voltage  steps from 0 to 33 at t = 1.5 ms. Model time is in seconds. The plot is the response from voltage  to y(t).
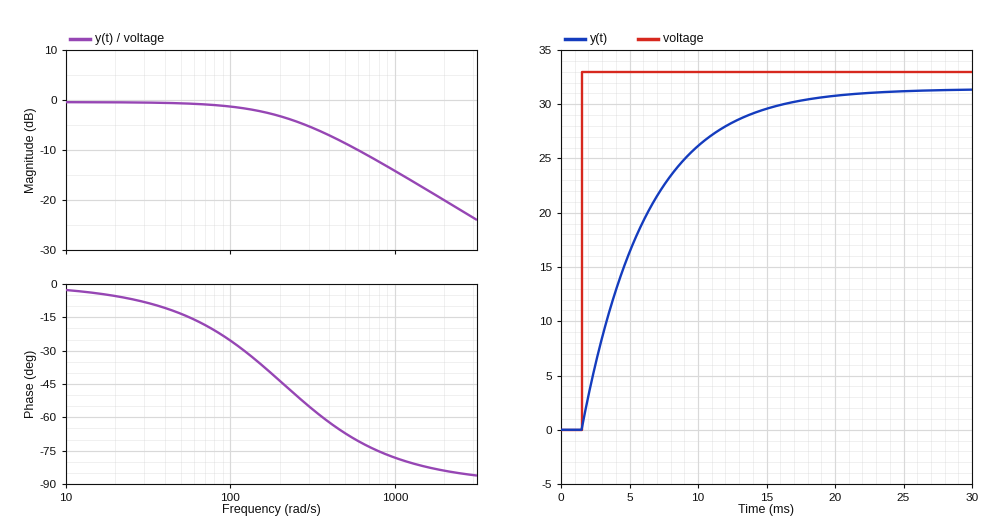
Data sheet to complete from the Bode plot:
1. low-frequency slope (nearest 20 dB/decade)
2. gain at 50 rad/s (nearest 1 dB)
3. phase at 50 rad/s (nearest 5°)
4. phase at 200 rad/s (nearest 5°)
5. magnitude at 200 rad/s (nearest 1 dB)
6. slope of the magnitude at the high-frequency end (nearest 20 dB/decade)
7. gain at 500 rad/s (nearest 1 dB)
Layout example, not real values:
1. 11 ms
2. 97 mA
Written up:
1. 0 dB/decade
2. -1 dB
3. -15°
4. -45°
5. -3 dB
6. -20 dB/decade
7. -9 dB
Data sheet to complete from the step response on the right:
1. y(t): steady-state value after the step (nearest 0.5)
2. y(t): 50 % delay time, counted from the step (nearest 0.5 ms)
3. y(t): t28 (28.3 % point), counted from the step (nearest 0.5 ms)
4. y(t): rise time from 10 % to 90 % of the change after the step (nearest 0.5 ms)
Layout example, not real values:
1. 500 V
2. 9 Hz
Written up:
1. 31.5
2. 3.5 ms
3. 1.5 ms
4. 10.5 ms
